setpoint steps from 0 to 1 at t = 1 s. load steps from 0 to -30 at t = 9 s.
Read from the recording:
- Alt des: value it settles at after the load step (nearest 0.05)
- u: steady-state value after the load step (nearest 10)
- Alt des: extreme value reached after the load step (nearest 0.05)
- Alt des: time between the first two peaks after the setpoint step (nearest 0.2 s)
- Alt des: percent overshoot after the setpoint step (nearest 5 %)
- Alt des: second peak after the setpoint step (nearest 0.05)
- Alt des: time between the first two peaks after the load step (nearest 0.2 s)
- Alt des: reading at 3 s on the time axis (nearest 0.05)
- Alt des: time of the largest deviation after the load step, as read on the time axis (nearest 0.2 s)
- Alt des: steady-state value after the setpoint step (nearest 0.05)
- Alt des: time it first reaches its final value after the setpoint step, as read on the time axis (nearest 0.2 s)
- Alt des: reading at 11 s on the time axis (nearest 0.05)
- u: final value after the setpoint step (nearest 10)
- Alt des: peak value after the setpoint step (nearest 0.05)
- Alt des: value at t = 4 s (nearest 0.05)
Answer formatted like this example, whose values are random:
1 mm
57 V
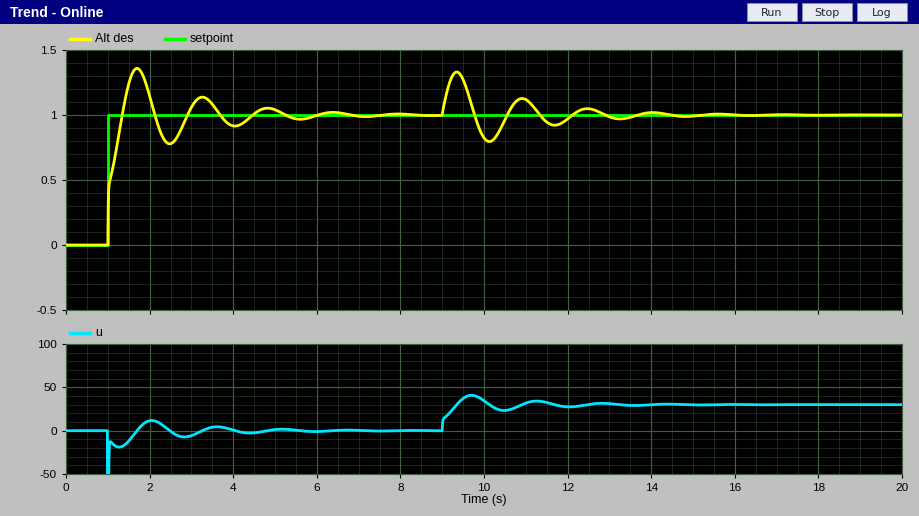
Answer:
1.00
30
1.35
1.6 s
35 %
1.15
1.6 s
1.05
9.4 s
1.00
1.4 s
1.10
0
1.35
0.90
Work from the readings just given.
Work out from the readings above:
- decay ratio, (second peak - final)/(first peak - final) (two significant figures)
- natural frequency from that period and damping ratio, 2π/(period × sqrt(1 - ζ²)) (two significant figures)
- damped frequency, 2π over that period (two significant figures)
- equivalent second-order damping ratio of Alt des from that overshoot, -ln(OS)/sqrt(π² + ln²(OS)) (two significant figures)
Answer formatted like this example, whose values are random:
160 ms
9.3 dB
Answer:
0.43
4.1 rad/s
3.9 rad/s
0.32
